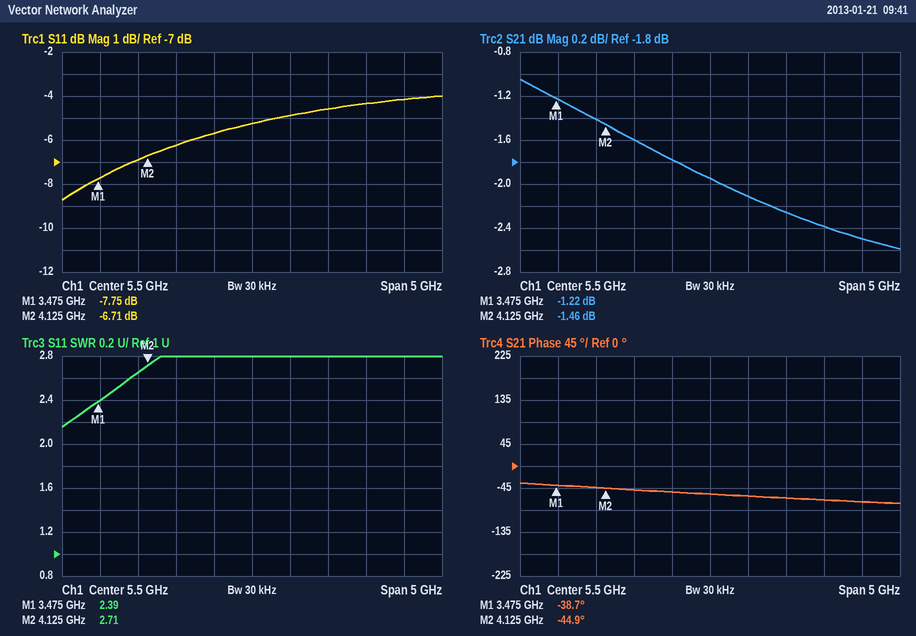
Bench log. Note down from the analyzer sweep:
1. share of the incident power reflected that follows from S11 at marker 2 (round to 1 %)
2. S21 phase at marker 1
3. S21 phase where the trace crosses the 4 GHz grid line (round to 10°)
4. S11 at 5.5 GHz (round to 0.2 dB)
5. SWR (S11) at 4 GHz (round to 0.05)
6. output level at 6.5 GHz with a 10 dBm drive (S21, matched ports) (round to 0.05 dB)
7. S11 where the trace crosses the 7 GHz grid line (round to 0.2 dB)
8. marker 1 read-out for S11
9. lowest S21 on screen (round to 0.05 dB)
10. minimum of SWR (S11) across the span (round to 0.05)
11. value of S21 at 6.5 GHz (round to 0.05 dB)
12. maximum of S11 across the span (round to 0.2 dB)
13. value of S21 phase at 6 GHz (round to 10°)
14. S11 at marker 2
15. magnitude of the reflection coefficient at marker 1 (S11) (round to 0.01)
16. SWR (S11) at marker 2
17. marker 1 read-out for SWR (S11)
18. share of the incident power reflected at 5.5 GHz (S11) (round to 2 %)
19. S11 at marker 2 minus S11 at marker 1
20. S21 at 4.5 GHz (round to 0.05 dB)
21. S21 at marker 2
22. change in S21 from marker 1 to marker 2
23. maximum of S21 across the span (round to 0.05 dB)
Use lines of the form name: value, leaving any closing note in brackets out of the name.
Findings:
share of the incident power reflected that follows from S11 at marker 2: 21 %
S21 phase at marker 1: -38.7°
S21 phase where the trace crosses the 4 GHz grid line: -40°
S11 at 5.5 GHz: -5.2 dB
SWR (S11) at 4 GHz: 2.65
output level at 6.5 GHz with a 10 dBm drive (S21, matched ports): 7.75 dBm
S11 where the trace crosses the 7 GHz grid line: -4.4 dB
marker 1 read-out for S11: -7.75 dB
lowest S21 on screen: -2.60 dB
minimum of SWR (S11) across the span: 2.15
value of S21 at 6.5 GHz: -2.25 dB
maximum of S11 across the span: -4.0 dB
value of S21 phase at 6 GHz: -60°
S11 at marker 2: -6.71 dB
magnitude of the reflection coefficient at marker 1 (S11): 0.41
SWR (S11) at marker 2: 2.71
marker 1 read-out for SWR: 2.39
share of the incident power reflected at 5.5 GHz (S11): 30 %
S11 at marker 2 minus S11 at marker 1: 1.04 dB
S21 at 4.5 GHz: -1.60 dB
S21 at marker 2: -1.46 dB
change in S21 from marker 1 to marker 2: -0.24 dB
maximum of S21 across the span: -1.05 dB
